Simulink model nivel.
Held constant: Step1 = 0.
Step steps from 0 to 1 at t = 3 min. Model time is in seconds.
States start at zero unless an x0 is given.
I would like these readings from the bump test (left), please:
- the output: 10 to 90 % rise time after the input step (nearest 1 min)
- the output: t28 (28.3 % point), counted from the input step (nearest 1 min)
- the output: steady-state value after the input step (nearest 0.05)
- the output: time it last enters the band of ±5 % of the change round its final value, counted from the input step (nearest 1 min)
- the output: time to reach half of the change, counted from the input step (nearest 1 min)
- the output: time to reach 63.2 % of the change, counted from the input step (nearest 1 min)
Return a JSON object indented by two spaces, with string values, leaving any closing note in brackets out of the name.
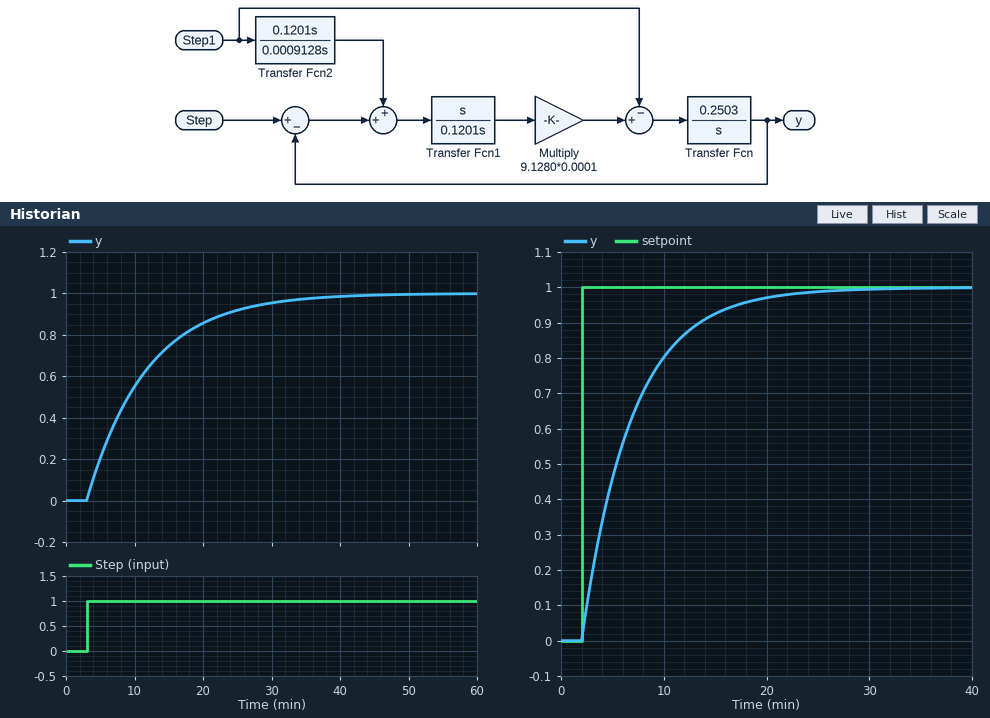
{
  "the output: 10 to 90 % rise time after the input step": "19 min",
  "the output: t28 (28.3 % point), counted from the input step": "3 min",
  "the output: steady-state value after the input step": "1.00",
  "the output: time it last enters the band of ±5 % of the change round its final value, counted from the input step": "26 min",
  "the output: time to reach half of the change, counted from the input step": "6 min",
  "the output: time to reach 63.2 % of the change, counted from the input step": "9 min"
}
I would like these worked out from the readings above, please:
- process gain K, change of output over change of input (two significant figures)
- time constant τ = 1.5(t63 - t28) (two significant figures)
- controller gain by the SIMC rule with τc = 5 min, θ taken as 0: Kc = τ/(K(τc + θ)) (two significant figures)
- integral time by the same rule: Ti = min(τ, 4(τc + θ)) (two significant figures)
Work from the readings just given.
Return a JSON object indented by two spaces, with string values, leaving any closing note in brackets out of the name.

{
  "process gain K, change of output over change of input": "1.0",
  "time constant τ = 1.5(t63 - t28)": "9.0 min",
  "controller gain by the SIMC rule with τc = 5 min, θ taken as 0: Kc = τ/(K(τc + θ))": "1.8",
  "integral time by the same rule: Ti = min(τ, 4(τc + θ))": "9.0 min"
}
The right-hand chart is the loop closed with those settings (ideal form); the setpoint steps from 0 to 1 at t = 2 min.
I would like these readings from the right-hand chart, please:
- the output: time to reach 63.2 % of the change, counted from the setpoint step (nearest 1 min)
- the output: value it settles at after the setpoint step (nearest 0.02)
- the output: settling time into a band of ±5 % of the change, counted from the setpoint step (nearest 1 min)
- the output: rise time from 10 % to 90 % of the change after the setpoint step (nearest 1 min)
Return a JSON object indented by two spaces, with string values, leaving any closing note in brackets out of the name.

{
  "the output: time to reach 63.2 % of the change, counted from the setpoint step": "5 min",
  "the output: value it settles at after the setpoint step": "1.00",
  "the output: settling time into a band of ±5 % of the change, counted from the setpoint step": "15 min",
  "the output: rise time from 10 % to 90 % of the change after the setpoint step": "11 min"
}
